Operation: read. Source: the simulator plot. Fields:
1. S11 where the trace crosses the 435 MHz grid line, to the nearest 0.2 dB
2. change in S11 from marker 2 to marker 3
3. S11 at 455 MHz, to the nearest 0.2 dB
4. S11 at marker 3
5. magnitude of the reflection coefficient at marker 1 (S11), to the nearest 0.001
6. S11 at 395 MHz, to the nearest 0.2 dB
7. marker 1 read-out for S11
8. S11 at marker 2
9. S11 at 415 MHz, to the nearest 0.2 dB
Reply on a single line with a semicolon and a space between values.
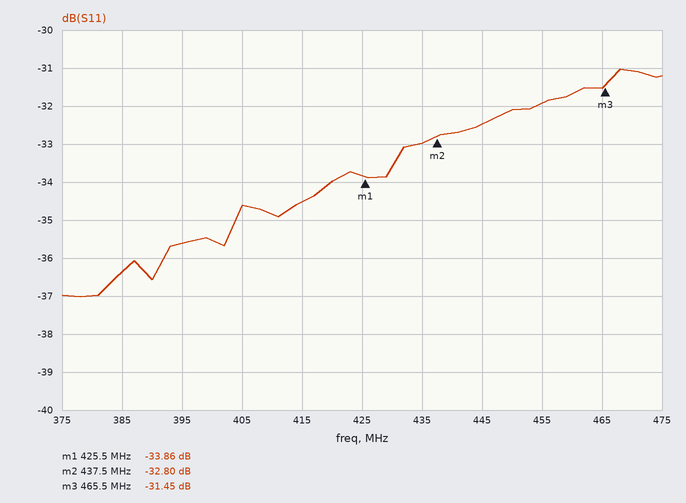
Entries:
-33.0 dB; 1.35 dB; -32.0 dB; -31.45 dB; 0.020; -35.6 dB; -33.86 dB; -32.80 dB; -34.6 dB
